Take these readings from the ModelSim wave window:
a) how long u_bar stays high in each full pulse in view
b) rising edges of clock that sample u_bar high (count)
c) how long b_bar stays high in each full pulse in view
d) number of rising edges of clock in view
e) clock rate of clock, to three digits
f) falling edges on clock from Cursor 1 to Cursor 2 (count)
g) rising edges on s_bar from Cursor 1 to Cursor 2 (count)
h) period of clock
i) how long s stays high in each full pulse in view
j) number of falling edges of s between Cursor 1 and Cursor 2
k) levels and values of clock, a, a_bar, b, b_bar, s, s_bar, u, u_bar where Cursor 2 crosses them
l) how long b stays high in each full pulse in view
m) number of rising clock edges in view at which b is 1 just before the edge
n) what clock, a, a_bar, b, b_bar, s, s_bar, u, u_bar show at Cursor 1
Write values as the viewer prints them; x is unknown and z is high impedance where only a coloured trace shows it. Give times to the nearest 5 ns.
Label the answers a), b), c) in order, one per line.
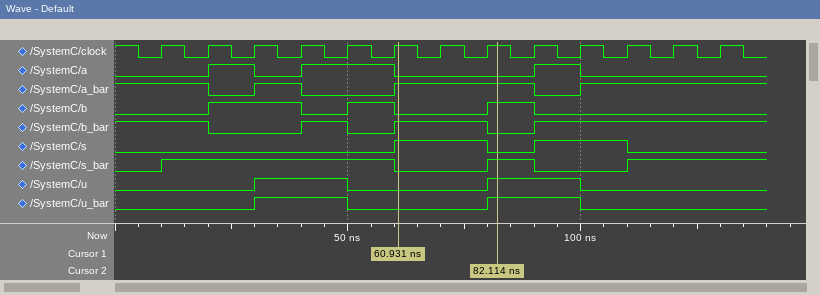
a) 20 ns, 20 ns
b) 4
c) 10 ns, 20 ns
d) 13
e) 100 MHz
f) 2
g) 1
h) 10 ns
i) 20 ns, 20 ns
j) 1
k) clock=1, a=0, a_bar=1, b=1, b_bar=0, s=0, s_bar=1, u=1, u_bar=1
l) 20 ns, 10 ns, 10 ns
m) 4
n) clock=1, a=0, a_bar=1, b=0, b_bar=1, s=1, s_bar=0, u=0, u_bar=0
